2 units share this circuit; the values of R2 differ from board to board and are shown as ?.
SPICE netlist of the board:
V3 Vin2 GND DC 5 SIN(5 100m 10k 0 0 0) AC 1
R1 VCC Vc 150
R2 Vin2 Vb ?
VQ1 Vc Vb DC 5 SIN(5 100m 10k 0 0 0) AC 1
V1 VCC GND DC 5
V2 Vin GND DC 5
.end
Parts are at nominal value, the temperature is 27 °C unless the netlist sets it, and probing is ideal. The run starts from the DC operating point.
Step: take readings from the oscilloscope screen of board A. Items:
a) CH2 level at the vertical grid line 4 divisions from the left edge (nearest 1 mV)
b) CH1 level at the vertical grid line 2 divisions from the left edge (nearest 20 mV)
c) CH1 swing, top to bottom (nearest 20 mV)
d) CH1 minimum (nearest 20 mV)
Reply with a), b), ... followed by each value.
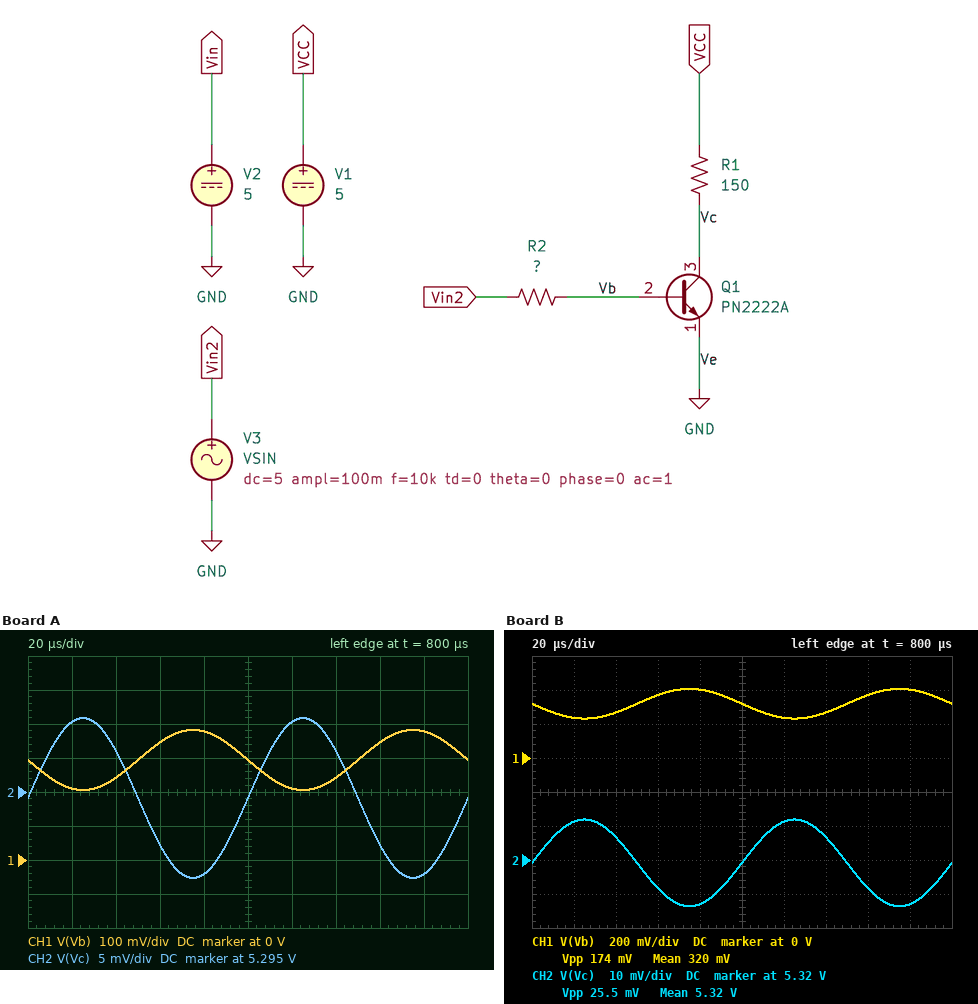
a) 5.283 V
b) 240 mV
c) 180 mV
d) 200 mV
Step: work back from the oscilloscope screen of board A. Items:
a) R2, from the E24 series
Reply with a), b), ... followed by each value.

a) 2.4 kΩ
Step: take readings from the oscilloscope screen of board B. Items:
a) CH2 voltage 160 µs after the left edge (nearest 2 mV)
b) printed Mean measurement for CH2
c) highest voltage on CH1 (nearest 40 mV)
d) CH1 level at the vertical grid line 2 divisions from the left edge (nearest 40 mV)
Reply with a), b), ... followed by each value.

a) 5.312 V
b) 5.32 V
c) 400 mV
d) 280 mV
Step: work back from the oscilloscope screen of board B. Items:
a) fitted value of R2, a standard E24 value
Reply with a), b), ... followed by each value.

a) 2.2 kΩ
